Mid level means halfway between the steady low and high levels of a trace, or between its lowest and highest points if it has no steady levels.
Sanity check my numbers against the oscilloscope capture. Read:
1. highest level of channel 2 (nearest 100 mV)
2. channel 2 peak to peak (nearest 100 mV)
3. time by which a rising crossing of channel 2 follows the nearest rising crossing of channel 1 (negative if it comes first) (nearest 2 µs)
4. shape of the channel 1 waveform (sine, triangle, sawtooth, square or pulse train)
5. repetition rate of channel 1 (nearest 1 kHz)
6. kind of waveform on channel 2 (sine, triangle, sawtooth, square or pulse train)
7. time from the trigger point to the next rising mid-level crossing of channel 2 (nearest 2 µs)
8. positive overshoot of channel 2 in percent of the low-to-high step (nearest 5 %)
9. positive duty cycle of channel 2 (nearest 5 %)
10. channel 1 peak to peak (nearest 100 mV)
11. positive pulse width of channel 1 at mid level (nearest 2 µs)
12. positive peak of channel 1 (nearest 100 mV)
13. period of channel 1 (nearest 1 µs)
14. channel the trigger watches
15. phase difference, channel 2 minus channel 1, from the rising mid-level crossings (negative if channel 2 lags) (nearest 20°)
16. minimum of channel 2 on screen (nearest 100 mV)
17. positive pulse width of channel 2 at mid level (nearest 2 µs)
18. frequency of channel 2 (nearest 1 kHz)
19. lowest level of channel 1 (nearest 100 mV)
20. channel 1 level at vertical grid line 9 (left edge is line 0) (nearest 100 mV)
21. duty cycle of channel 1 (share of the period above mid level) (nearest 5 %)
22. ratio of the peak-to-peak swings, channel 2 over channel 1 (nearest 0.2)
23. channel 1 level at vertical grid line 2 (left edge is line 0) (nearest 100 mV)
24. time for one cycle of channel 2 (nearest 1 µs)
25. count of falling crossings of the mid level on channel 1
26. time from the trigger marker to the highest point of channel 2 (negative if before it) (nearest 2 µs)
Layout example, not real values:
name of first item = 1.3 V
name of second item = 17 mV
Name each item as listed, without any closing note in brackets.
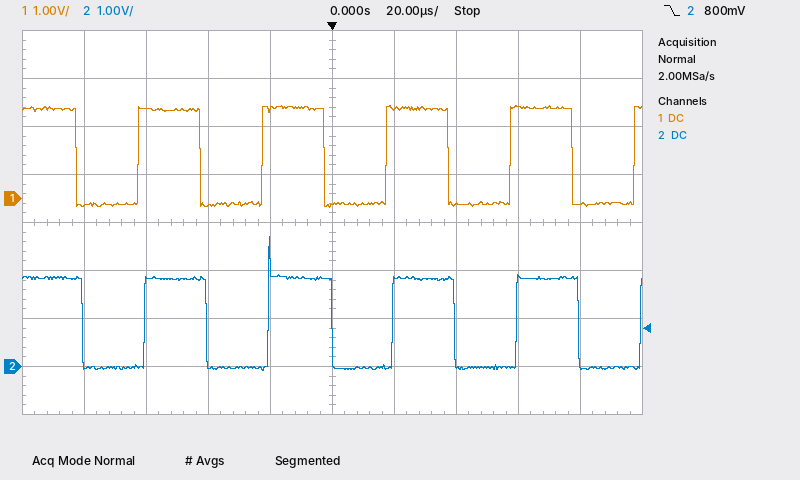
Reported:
highest level of channel 2 = 2.7 V
channel 2 peak to peak = 2.8 V
time by which a rising crossing of channel 2 follows the nearest rising crossing of channel 1 (negative if it comes first) = +2 µs
shape of the channel 1 waveform = square
repetition rate of channel 1 = 25 kHz
kind of waveform on channel 2 = square
time from the trigger point to the next rising mid-level crossing of channel 2 = 20 µs
positive overshoot of channel 2 in percent of the low-to-high step = 45 %
positive duty cycle of channel 2 = 50 %
channel 1 peak to peak = 2.1 V
positive pulse width of channel 1 at mid level = 20 µs
positive peak of channel 1 = 1.9 V
period of channel 1 = 40 µs
channel the trigger watches = channel 2
phase difference, channel 2 minus channel 1, from the rising mid-level crossings (negative if channel 2 lags) = -20°
minimum of channel 2 on screen = -100 mV
positive pulse width of channel 2 at mid level = 20 µs
frequency of channel 2 = 25 kHz
lowest level of channel 1 = -200 mV
channel 1 level at vertical grid line 9 (left edge is line 0) = -100 mV
duty cycle of channel 1 (share of the period above mid level) = 50 %
ratio of the peak-to-peak swings, channel 2 over channel 1 = 1.4
channel 1 level at vertical grid line 2 (left edge is line 0) = 1.9 V
time for one cycle of channel 2 = 40 µs
count of falling crossings of the mid level on channel 1 = 5
time from the trigger marker to the highest point of channel 2 (negative if before it) = -20 µs
